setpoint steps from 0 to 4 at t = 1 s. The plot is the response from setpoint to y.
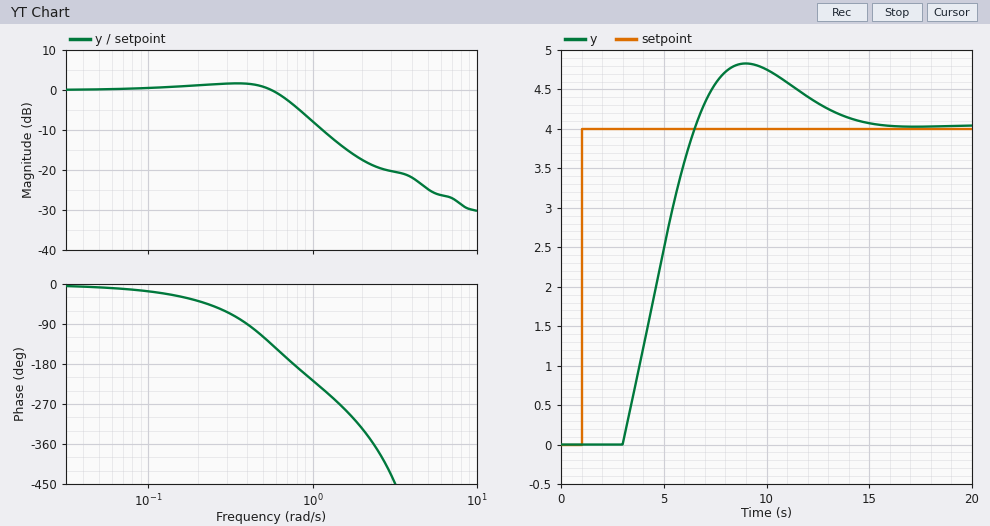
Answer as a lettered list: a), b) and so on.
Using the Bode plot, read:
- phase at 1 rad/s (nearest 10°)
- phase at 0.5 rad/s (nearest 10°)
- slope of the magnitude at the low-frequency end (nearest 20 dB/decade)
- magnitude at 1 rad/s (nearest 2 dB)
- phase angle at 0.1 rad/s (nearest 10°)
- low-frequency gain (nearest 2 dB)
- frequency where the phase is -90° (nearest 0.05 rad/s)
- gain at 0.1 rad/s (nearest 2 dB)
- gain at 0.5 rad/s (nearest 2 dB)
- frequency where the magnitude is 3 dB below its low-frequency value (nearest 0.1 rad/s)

a) -220°
b) -120°
c) 0 dB/decade
d) -8 dB
e) -20°
f) 0 dB
g) 0.40 rad/s
h) 0 dB
i) 0 dB
j) 0.7 rad/s
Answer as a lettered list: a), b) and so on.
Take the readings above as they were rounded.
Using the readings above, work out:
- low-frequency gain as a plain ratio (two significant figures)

a) 1.0
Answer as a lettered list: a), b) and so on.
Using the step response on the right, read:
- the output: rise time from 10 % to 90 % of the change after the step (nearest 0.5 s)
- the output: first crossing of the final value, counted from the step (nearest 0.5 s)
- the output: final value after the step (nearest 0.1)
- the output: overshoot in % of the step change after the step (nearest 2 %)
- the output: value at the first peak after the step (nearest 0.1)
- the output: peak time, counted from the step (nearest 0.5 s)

a) 2.5 s
b) 5.5 s
c) 4.0
d) 20 %
e) 4.8
f) 8.0 s
